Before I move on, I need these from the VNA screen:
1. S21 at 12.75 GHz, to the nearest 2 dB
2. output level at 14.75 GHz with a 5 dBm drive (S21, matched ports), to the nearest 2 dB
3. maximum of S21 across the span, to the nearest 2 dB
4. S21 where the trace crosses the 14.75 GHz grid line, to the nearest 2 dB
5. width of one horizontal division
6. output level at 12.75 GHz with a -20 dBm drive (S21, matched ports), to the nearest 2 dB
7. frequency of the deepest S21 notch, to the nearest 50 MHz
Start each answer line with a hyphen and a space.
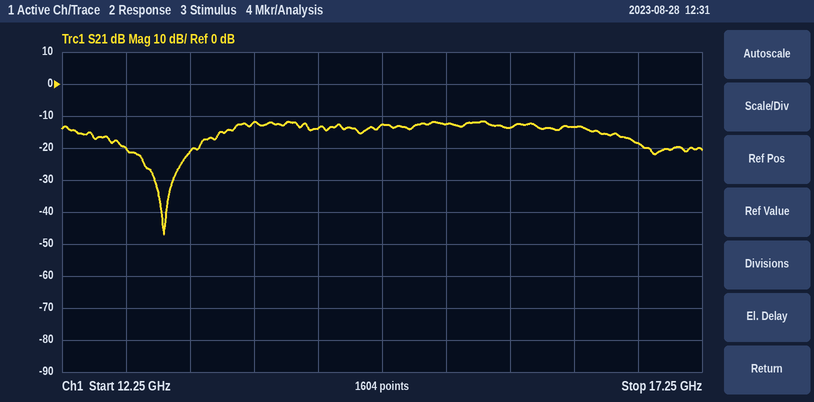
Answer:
- -20 dB
- -8 dBm
- -12 dB
- -12 dB
- 500 MHz
- -40 dBm
- 13.05 GHz
